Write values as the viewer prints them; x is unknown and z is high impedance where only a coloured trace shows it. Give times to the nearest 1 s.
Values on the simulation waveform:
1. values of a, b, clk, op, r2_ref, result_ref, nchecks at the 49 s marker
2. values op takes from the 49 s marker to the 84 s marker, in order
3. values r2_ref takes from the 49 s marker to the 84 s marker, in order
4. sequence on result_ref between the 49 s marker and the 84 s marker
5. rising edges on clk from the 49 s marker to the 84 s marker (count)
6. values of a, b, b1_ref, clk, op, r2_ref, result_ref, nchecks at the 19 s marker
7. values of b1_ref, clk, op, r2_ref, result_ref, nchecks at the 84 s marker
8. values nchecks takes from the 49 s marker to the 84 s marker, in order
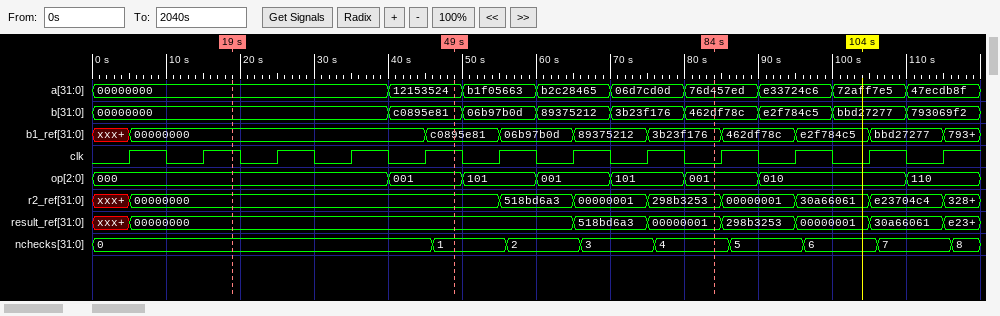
a=12153524, b=c0895e81, clk=1, op=001, r2_ref=00000000, result_ref=00000000, nchecks=1
001, 101, 001, 101, 001
00000000, 518bd6a3, 00000001, 298b3253
00000000, 518bd6a3, 00000001
3
a=00000000, b=00000000, b1_ref=00000000, clk=1, op=000, r2_ref=00000000, result_ref=00000000, nchecks=0
b1_ref=3b23f176, clk=0, op=001, r2_ref=298b3253, result_ref=00000001, nchecks=4
1, 2, 3, 4
